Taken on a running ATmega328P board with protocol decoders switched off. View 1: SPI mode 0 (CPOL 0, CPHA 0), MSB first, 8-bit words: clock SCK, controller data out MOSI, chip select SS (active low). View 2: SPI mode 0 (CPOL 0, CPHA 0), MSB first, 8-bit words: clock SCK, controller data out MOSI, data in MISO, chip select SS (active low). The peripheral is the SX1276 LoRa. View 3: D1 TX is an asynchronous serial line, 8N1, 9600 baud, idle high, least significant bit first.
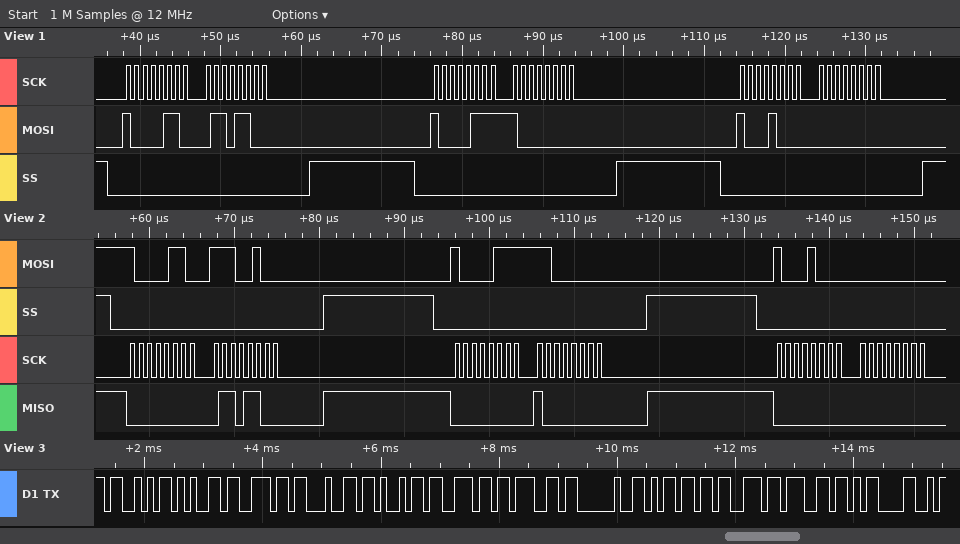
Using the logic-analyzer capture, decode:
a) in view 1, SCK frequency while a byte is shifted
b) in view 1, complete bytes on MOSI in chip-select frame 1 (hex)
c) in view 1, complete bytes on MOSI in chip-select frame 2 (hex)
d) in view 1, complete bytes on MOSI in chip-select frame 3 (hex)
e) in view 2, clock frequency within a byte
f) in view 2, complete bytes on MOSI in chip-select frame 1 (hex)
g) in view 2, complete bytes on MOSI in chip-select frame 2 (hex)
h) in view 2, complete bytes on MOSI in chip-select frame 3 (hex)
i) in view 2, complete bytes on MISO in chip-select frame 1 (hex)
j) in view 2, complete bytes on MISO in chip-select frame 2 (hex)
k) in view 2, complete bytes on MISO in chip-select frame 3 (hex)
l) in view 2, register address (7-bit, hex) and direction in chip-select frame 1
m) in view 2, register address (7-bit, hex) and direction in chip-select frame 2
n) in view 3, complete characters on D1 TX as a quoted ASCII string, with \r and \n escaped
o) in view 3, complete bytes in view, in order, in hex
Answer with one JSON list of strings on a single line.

["1 MHz", "86 6C", "87 80", "88 00", "1 MHz", "0x86 0xE4", "0x87 0xC0", "0x88 0x00", "0x00 0x6C", "0x00 0x80", "0x00 0x00", "0x06 write", "0x07 write", "\"Sending msg\\r\"", "53 65 6E 64 69 6E 67 20 6D 73 67 0D"]
